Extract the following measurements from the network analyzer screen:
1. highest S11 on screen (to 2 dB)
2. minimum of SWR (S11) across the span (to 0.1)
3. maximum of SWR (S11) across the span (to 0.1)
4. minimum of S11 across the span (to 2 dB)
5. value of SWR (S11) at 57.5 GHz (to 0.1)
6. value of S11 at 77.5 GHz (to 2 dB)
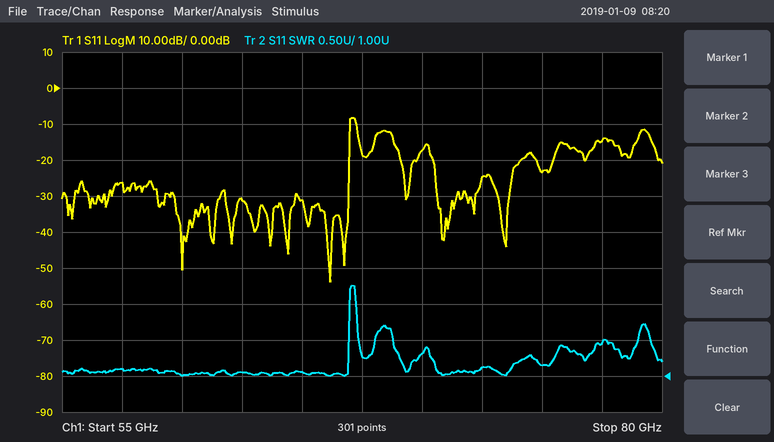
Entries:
-8 dB
1.0
2.3
-54 dB
1.1
-14 dB
